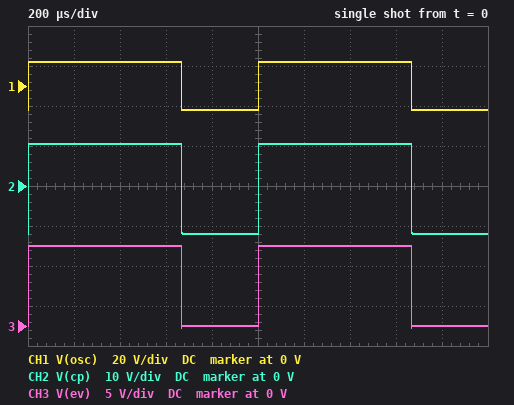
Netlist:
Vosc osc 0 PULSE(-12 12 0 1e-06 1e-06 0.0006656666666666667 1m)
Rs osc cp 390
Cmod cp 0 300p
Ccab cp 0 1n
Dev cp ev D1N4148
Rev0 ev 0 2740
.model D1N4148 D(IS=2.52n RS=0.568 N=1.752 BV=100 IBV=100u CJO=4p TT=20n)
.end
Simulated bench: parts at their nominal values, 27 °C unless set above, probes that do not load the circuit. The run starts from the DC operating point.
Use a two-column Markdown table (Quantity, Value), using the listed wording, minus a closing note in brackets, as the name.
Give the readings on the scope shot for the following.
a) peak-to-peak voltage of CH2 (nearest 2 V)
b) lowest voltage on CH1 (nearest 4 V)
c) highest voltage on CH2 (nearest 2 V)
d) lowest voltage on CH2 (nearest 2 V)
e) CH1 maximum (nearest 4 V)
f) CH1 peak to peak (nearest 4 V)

| Quantity | Value |
|---|---|
| peak-to-peak voltage of CH2 | 22 V |
| lowest voltage on CH1 | -12 V |
| highest voltage on CH2 | 10 V |
| lowest voltage on CH2 | -12 V |
| CH1 maximum | 12 V |
| CH1 peak to peak | 24 V |
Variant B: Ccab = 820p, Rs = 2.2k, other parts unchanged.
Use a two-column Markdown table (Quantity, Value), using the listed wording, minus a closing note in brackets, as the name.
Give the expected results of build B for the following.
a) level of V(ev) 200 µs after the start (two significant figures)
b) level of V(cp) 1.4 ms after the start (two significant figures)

| Quantity | Value |
|---|---|
| level of V(ev) 200 µs after the start | 6.3 V |
| level of V(cp) 1.4 ms after the start | 6.9 V |
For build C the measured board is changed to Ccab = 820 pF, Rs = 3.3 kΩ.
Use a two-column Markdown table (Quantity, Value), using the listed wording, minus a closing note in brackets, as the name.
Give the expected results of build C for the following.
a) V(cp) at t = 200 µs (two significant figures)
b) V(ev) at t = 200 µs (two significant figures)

| Quantity | Value |
|---|---|
| V(cp) at t = 200 µs | 5.8 V |
| V(ev) at t = 200 µs | 5.2 V |
